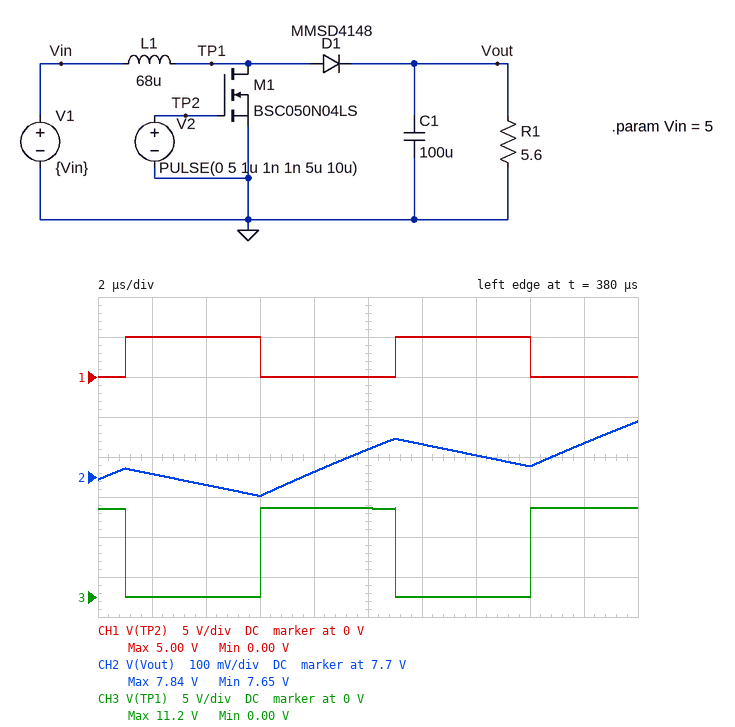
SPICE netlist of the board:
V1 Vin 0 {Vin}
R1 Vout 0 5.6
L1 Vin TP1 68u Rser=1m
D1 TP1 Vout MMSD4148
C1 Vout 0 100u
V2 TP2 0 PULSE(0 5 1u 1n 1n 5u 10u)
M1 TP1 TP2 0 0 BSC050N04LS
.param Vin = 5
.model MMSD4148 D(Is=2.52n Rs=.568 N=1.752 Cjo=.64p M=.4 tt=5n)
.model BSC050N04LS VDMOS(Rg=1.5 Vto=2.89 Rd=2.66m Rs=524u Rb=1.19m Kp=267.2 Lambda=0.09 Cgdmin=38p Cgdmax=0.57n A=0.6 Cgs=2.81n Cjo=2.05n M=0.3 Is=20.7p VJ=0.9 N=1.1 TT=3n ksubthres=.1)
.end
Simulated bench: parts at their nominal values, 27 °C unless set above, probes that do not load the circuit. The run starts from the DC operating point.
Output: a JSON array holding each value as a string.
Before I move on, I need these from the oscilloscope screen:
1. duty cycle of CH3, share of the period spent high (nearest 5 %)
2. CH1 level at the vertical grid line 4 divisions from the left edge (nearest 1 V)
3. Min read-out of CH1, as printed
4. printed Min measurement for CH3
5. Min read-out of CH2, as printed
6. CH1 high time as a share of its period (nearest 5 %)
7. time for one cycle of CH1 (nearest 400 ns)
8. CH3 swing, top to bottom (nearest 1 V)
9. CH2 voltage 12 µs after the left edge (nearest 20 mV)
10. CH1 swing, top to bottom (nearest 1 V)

["50 %", "0 V", "0.00 V", "0.00 V", "7.65 V", "50 %", "10.0 µs", "11 V", "7.78 V", "5 V"]
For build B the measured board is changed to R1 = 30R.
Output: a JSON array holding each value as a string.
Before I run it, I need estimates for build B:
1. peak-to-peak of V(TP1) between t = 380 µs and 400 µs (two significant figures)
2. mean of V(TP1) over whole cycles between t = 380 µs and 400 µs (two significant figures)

["12 V", "5.9 V"]
